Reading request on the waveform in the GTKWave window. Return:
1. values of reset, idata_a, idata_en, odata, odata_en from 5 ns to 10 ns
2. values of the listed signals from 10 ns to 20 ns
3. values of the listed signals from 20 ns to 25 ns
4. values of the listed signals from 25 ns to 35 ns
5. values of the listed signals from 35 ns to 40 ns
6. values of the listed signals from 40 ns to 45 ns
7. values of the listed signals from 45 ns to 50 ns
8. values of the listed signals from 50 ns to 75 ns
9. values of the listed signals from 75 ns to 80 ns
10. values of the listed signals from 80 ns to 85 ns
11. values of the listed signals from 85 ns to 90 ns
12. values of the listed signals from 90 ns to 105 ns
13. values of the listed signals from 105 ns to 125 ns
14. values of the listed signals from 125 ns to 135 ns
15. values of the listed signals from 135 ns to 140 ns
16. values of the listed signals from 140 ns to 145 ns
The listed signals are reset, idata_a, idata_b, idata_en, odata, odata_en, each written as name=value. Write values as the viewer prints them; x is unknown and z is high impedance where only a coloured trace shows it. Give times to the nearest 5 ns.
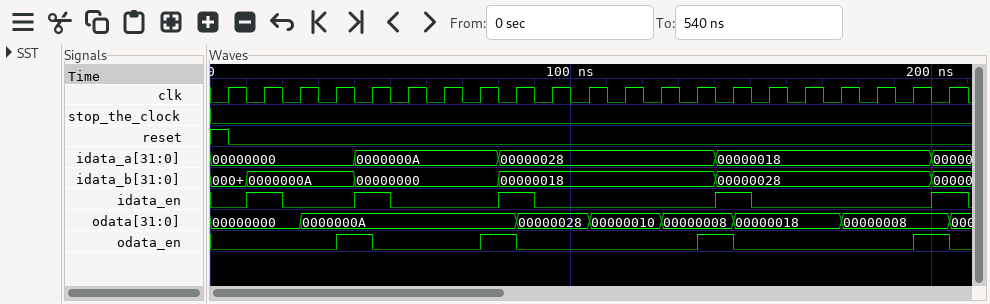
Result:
reset=0, idata_a=00000000, idata_en=0, odata=00000000, odata_en=0
reset=0, idata_a=00000000, idata_b=0000000A, idata_en=1, odata=00000000, odata_en=0
reset=0, idata_a=00000000, idata_b=0000000A, idata_en=0, odata=00000000, odata_en=0
reset=0, idata_a=00000000, idata_b=0000000A, idata_en=0, odata=0000000A, odata_en=0
reset=0, idata_a=00000000, idata_b=0000000A, idata_en=0, odata=0000000A, odata_en=1
reset=0, idata_a=0000000A, idata_b=00000000, idata_en=1, odata=0000000A, odata_en=1
reset=0, idata_a=0000000A, idata_b=00000000, idata_en=1, odata=0000000A, odata_en=0
reset=0, idata_a=0000000A, idata_b=00000000, idata_en=0, odata=0000000A, odata_en=0
reset=0, idata_a=0000000A, idata_b=00000000, idata_en=0, odata=0000000A, odata_en=1
reset=0, idata_a=00000028, idata_b=00000018, idata_en=1, odata=0000000A, odata_en=1
reset=0, idata_a=00000028, idata_b=00000018, idata_en=1, odata=00000028, odata_en=0
reset=0, idata_a=00000028, idata_b=00000018, idata_en=0, odata=00000028, odata_en=0
reset=0, idata_a=00000028, idata_b=00000018, idata_en=0, odata=00000010, odata_en=0
reset=0, idata_a=00000028, idata_b=00000018, idata_en=0, odata=00000008, odata_en=0
reset=0, idata_a=00000028, idata_b=00000018, idata_en=0, odata=00000008, odata_en=1
reset=0, idata_a=00000018, idata_b=00000028, idata_en=1, odata=00000008, odata_en=1
